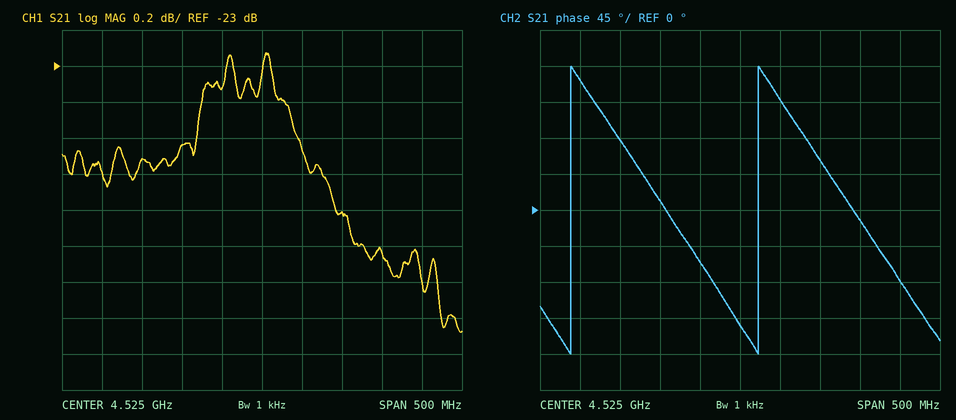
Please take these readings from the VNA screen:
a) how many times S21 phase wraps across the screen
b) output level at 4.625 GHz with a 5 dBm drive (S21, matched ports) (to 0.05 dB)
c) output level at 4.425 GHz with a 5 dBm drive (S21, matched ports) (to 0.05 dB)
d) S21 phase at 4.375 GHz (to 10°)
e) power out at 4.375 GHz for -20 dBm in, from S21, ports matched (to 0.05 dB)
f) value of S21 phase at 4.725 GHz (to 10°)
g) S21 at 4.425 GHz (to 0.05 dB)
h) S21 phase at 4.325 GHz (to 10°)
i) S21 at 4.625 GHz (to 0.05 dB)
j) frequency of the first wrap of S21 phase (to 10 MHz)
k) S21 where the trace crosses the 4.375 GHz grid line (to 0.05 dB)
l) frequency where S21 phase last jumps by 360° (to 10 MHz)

2
-18.80 dBm
-18.45 dBm
90°
-43.50 dBm
-90°
-23.45 dB
160°
-23.80 dB
4.31 GHz
-23.50 dB
4.55 GHz
